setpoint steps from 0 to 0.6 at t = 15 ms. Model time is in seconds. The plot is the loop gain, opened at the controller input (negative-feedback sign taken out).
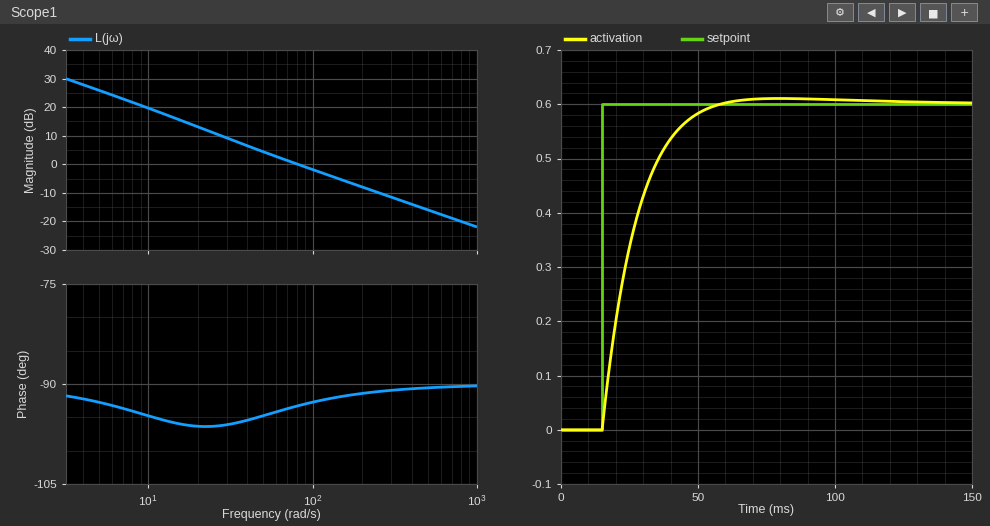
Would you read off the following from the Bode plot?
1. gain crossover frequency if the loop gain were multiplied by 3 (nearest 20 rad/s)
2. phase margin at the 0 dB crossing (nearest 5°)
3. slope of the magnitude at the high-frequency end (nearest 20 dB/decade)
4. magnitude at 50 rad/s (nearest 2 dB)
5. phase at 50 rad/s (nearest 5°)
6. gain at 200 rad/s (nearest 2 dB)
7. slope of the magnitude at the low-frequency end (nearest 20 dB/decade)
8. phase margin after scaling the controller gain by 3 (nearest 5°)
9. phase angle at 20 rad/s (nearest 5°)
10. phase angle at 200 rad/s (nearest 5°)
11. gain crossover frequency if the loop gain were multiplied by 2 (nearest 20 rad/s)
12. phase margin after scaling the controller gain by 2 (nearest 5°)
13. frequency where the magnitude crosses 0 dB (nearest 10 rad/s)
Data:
240 rad/s
85°
-20 dB/decade
4 dB
-95°
-8 dB
-20 dB/decade
90°
-95°
-90°
160 rad/s
90°
80 rad/s
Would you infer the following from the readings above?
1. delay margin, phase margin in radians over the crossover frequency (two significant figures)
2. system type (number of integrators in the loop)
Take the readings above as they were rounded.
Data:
0.019 s
1
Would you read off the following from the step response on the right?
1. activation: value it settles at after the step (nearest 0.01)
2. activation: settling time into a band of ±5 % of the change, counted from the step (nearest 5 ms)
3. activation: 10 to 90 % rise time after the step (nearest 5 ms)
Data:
0.60
30 ms
25 ms
